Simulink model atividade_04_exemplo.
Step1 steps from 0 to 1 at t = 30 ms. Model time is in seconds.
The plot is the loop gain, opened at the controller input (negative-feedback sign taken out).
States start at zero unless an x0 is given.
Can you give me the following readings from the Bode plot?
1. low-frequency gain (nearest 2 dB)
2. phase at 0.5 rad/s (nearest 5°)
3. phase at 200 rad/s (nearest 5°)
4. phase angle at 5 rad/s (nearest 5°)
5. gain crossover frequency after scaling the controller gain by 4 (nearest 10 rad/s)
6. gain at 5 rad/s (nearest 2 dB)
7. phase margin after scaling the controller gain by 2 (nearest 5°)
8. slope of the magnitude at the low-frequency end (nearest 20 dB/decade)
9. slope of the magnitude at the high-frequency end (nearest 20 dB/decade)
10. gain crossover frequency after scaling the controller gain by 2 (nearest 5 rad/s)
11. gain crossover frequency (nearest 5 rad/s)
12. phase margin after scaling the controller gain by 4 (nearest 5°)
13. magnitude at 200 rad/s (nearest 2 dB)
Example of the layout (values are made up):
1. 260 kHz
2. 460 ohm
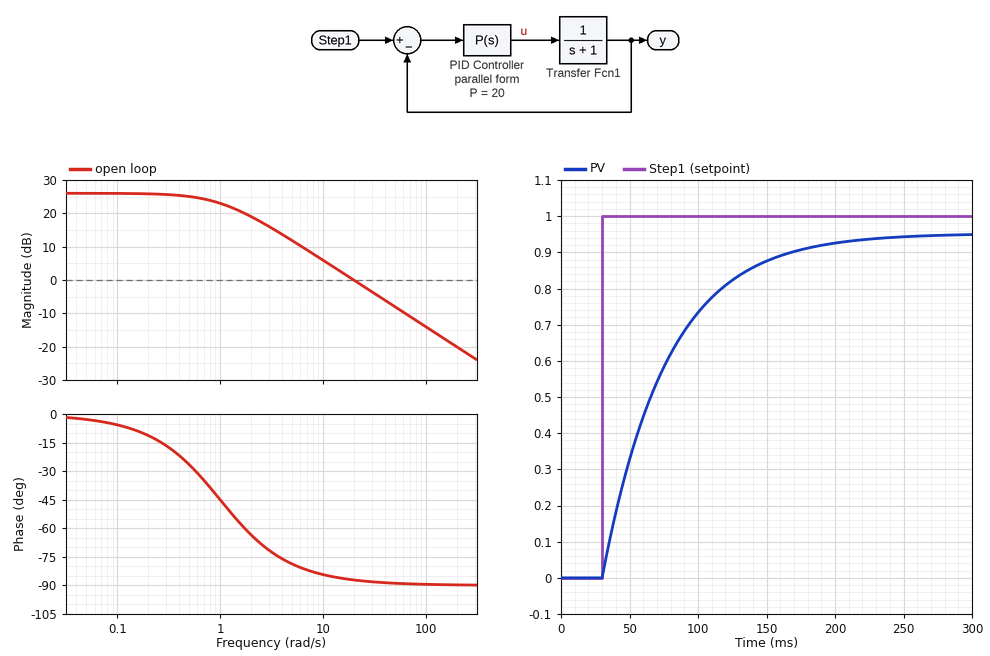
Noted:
1. 26 dB
2. -25°
3. -90°
4. -80°
5. 80 rad/s
6. 12 dB
7. 90°
8. 0 dB/decade
9. -20 dB/decade
10. 40 rad/s
11. 20 rad/s
12. 90°
13. -20 dB
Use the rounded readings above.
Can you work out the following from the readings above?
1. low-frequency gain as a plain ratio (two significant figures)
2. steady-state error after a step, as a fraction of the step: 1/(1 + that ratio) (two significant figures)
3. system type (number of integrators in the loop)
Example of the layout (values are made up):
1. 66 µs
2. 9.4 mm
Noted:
1. 20
2. 0.048
3. 0
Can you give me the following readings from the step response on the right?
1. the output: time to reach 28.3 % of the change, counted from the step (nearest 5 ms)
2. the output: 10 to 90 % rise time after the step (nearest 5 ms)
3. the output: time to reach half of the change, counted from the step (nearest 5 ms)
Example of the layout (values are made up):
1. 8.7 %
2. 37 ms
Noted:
1. 15 ms
2. 105 ms
3. 35 ms
